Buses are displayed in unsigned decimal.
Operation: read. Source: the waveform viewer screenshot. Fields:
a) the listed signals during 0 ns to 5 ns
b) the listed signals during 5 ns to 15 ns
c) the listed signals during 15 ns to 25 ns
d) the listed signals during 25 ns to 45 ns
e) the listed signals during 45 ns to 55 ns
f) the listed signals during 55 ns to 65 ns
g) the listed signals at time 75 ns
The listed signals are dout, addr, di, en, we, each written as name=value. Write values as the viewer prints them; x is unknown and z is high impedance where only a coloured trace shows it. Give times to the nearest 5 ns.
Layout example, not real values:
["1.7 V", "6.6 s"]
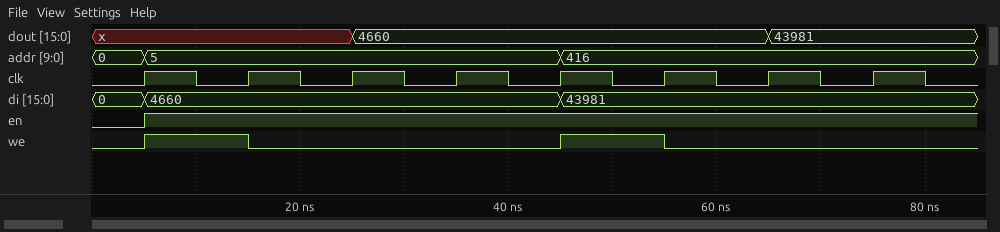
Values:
["dout=x, addr=0, di=0, en=0, we=0", "dout=x, addr=5, di=4660, en=1, we=1", "dout=x, addr=5, di=4660, en=1, we=0", "dout=4660, addr=5, di=4660, en=1, we=0", "dout=4660, addr=416, di=43981, en=1, we=1", "dout=4660, addr=416, di=43981, en=1, we=0", "dout=43981, addr=416, di=43981, en=1, we=0"]
